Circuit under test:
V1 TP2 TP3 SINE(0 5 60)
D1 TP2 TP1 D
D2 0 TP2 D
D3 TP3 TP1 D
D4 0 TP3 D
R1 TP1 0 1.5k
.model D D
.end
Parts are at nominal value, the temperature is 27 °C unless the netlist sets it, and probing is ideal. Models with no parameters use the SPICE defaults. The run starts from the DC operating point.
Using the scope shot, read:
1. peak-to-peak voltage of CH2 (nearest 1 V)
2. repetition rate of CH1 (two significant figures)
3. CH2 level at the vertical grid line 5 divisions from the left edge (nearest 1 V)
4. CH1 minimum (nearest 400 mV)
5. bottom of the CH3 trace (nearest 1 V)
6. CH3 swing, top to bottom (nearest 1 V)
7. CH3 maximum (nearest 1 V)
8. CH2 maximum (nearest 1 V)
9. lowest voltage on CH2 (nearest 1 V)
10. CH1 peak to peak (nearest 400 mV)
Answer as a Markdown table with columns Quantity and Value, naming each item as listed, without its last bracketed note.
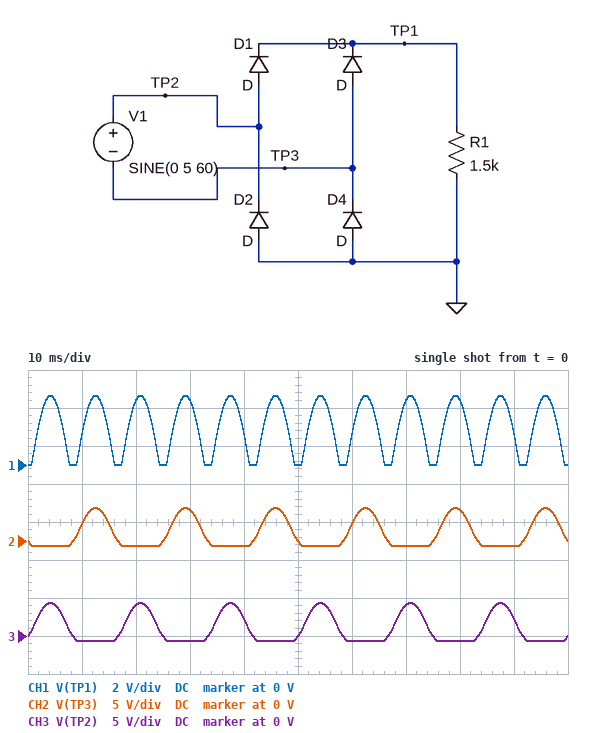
| Quantity | Value |
|---|---|
| peak-to-peak voltage of CH2 | 5 V |
| repetition rate of CH1 | 120 Hz |
| CH2 level at the vertical grid line 5 divisions from the left edge | 0 V |
| CH1 minimum | 0 V |
| bottom of the CH3 trace | -1 V |
| CH3 swing, top to bottom | 5 V |
| CH3 maximum | 4 V |
| CH2 maximum | 4 V |
| lowest voltage on CH2 | -1 V |
| CH1 peak to peak | 3.6 V |
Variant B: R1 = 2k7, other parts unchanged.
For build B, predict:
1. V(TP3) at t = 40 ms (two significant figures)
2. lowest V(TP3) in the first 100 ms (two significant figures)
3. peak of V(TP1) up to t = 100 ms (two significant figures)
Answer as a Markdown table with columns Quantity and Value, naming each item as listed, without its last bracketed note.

| Quantity | Value |
|---|---|
| V(TP3) at t = 40 ms | -640 mV |
| lowest V(TP3) in the first 100 ms | -660 mV |
| peak of V(TP1) up to t = 100 ms | 3.7 V |
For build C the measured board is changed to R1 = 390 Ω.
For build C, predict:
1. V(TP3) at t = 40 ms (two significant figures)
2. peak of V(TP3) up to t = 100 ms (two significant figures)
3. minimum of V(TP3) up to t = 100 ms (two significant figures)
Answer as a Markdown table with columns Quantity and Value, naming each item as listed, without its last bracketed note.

| Quantity | Value |
|---|---|
| V(TP3) at t = 40 ms | -690 mV |
| peak of V(TP3) up to t = 100 ms | 4.3 V |
| minimum of V(TP3) up to t = 100 ms | -710 mV |
